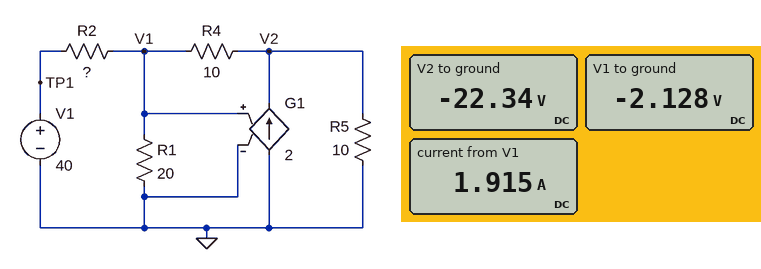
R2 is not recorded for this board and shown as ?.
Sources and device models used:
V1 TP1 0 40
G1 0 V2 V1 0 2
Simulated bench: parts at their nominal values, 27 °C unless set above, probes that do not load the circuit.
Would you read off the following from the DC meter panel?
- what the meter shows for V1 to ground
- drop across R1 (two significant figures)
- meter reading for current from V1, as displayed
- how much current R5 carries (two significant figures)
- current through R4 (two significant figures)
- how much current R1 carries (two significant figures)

-2.128 V
2.1 V
1.915 A
2.2 A
2.0 A
110 mA
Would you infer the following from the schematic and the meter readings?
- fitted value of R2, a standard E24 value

22 Ω
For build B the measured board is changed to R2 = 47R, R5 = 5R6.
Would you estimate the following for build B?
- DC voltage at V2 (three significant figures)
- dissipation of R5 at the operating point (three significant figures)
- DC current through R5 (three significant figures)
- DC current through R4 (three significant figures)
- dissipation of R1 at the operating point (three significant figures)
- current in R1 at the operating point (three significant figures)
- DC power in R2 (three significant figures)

-11.0 V
21.7 W
1.97 A
955 mA
107 mW
73.0 mA
36.6 W
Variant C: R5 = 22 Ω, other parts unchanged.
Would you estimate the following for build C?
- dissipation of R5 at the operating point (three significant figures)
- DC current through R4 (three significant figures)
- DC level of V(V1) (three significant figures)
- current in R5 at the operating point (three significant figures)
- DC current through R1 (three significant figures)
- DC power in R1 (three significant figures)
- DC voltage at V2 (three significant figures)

20.1 W
1.96 A
-1.46 V
956 mA
72.8 mA
106 mW
-21.0 V
